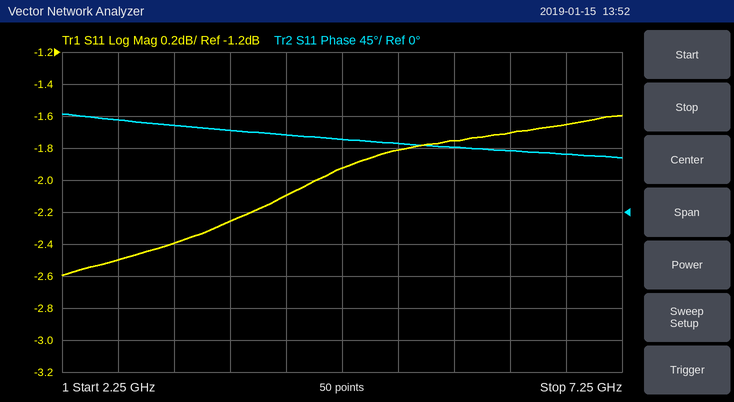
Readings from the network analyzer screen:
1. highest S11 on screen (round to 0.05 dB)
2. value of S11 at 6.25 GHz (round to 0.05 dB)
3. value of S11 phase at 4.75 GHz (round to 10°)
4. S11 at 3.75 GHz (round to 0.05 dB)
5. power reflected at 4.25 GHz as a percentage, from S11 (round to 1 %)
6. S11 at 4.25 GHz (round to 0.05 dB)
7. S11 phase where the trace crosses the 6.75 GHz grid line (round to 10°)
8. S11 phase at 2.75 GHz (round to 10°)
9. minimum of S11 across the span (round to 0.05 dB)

-1.60 dB
-1.70 dB
100°
-2.25 dB
62 %
-2.10 dB
80°
130°
-2.60 dB
